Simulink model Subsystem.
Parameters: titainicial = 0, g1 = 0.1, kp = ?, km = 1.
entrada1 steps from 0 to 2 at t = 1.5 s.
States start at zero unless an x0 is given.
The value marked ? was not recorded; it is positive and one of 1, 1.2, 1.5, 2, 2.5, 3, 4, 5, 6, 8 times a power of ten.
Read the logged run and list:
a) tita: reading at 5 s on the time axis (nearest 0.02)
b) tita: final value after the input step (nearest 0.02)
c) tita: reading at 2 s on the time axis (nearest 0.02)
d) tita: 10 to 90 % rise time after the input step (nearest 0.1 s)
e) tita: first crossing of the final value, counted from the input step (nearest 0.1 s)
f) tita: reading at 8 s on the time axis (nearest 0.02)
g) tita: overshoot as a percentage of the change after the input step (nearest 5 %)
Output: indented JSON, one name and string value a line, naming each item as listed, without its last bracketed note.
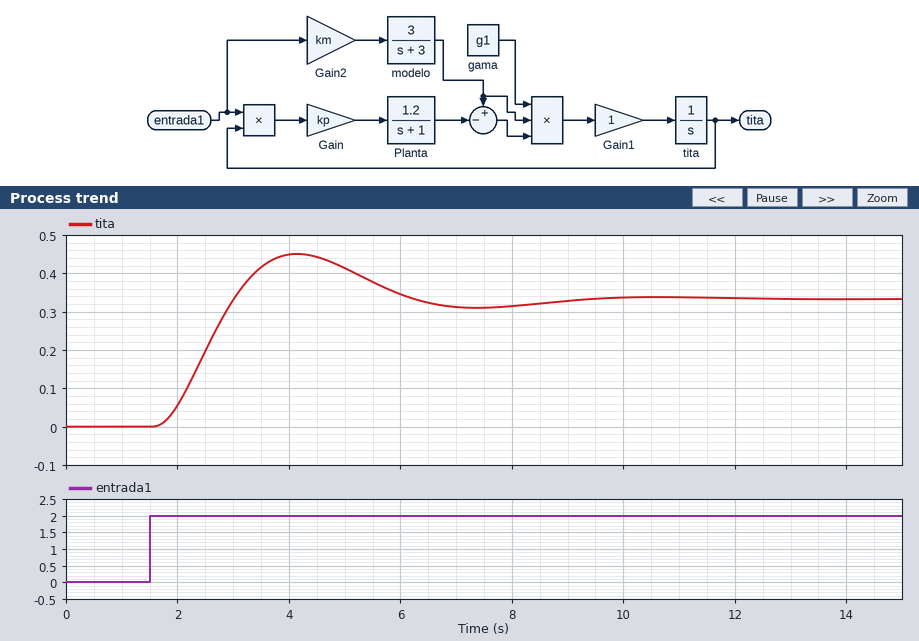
{
  "tita: reading at 5 s on the time axis": "0.42",
  "tita: final value after the input step": "0.34",
  "tita: reading at 2 s on the time axis": "0.06",
  "tita: 10 to 90 % rise time after the input step": "1.0 s",
  "tita: first crossing of the final value, counted from the input step": "1.5 s",
  "tita: reading at 8 s on the time axis": "0.32",
  "tita: overshoot as a percentage of the change after the input step": "35 %"
}
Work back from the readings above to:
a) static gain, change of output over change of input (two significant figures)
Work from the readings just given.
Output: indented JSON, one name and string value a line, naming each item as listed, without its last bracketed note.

{
  "static gain, change of output over change of input": "0.17"
}
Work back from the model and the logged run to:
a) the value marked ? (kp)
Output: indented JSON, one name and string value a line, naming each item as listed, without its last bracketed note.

{
  "the value marked ?": "2.5"
}
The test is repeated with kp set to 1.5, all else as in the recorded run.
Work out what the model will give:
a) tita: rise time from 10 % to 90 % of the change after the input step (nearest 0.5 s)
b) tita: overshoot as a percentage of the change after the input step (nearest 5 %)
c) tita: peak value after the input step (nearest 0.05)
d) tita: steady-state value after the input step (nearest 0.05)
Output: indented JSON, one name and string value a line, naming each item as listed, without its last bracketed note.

{
  "tita: rise time from 10 % to 90 % of the change after the input step": "1.5 s",
  "tita: overshoot as a percentage of the change after the input step": "15 %",
  "tita: peak value after the input step": "0.65",
  "tita: steady-state value after the input step": "0.55"
}
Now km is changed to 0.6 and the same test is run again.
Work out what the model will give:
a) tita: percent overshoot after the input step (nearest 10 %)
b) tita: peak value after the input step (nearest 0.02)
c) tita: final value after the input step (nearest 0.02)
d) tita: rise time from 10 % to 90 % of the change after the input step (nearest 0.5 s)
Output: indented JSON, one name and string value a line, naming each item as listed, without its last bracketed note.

{
  "tita: percent overshoot after the input step": "20 %",
  "tita: peak value after the input step": "0.24",
  "tita: final value after the input step": "0.20",
  "tita: rise time from 10 % to 90 % of the change after the input step": "1.5 s"
}
